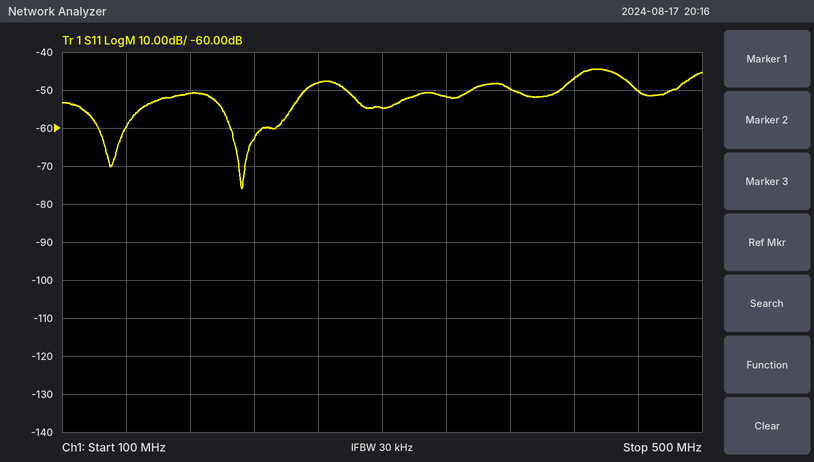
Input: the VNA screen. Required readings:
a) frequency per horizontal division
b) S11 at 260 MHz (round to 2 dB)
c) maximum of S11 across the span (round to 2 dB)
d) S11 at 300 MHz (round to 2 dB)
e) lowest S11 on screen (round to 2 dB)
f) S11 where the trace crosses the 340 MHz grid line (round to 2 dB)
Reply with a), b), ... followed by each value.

a) 40 MHz
b) -48 dB
c) -44 dB
d) -54 dB
e) -76 dB
f) -52 dB
